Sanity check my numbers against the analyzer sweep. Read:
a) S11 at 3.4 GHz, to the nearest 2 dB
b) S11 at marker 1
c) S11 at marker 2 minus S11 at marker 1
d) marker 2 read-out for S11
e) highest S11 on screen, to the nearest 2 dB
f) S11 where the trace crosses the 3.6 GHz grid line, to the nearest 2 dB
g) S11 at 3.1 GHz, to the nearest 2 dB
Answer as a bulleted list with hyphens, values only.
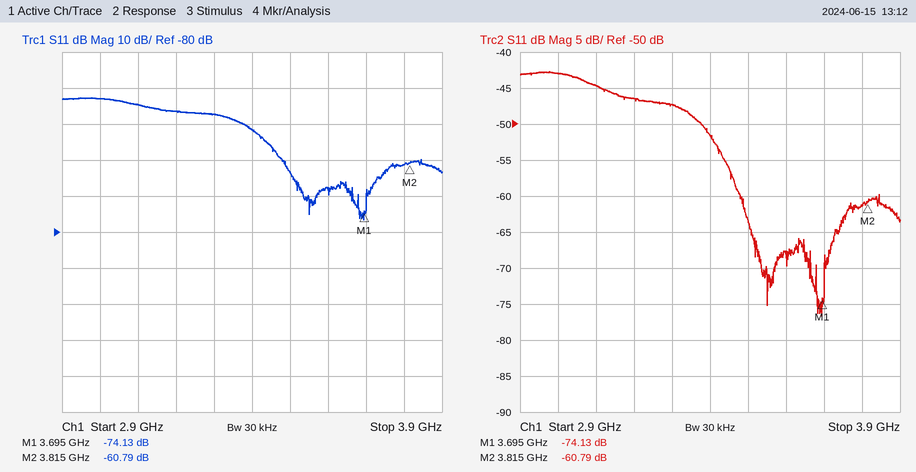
- -52 dB
- -74.13 dB
- 13.34 dB
- -60.79 dB
- -42 dB
- -68 dB
- -44 dB
